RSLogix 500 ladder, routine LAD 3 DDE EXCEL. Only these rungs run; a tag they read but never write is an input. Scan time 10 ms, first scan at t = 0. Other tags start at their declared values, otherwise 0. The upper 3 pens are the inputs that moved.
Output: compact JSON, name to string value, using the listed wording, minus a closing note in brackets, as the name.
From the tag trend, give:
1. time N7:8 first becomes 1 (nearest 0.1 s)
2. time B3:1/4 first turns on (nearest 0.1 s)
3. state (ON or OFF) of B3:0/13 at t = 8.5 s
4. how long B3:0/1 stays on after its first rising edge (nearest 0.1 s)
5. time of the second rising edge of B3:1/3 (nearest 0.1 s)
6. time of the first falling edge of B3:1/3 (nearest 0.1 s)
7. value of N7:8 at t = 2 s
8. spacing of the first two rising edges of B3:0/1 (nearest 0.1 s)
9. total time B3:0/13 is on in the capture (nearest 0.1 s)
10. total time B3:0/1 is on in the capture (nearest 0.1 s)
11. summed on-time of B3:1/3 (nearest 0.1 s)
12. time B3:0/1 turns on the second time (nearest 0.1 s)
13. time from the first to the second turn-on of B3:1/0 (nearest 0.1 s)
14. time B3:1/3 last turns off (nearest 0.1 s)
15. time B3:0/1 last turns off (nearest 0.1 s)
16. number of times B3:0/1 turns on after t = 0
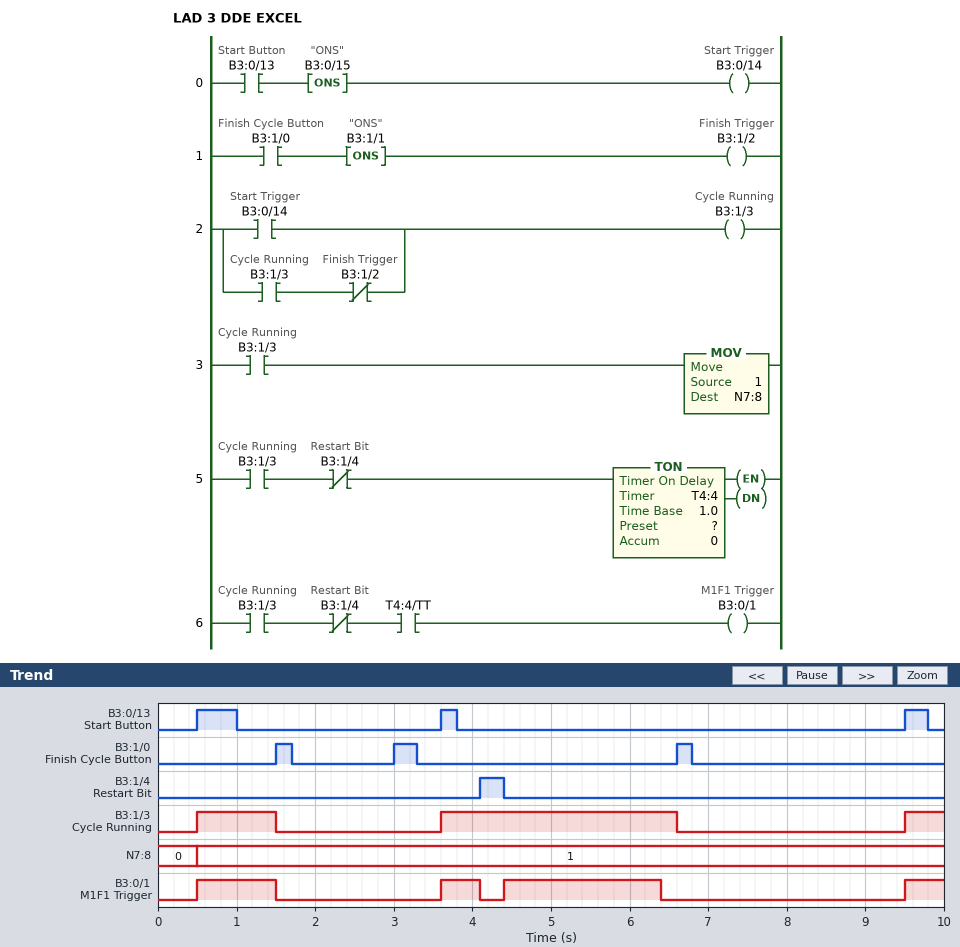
{"time N7:8 first becomes 1": "0.5 s", "time B3:1/4 first turns on": "4.1 s", "state (ON or OFF) of B3:0/13 at t = 8.5 s": "OFF", "how long B3:0/1 stays on after its first rising edge": "1.0 s", "time of the second rising edge of B3:1/3": "3.6 s", "time of the first falling edge of B3:1/3": "1.5 s", "value of N7:8 at t = 2 s": "1", "spacing of the first two rising edges of B3:0/1": "3.1 s", "total time B3:0/13 is on in the capture": "1.0 s", "total time B3:0/1 is on in the capture": "4.0 s", "summed on-time of B3:1/3": "4.5 s", "time B3:0/1 turns on the second time": "3.6 s", "time from the first to the second turn-on of B3:1/0": "1.5 s", "time B3:1/3 last turns off": "6.6 s", "time B3:0/1 last turns off": "6.4 s", "number of times B3:0/1 turns on after t = 0": "4"}
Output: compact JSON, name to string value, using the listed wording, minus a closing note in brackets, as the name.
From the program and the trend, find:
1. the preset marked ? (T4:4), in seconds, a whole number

{"the preset marked ? (T4:4), in seconds, a whole number": "2 s"}
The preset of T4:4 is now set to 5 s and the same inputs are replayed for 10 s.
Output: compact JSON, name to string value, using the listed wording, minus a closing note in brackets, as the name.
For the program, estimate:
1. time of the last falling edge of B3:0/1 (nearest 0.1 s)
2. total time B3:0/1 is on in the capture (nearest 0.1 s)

{"time of the last falling edge of B3:0/1": "6.6 s", "total time B3:0/1 is on in the capture": "4.2 s"}
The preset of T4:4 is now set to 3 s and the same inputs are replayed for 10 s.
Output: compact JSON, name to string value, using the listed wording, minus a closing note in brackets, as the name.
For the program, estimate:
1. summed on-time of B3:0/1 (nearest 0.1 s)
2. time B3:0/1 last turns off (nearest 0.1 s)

{"summed on-time of B3:0/1": "4.2 s", "time B3:0/1 last turns off": "6.6 s"}
